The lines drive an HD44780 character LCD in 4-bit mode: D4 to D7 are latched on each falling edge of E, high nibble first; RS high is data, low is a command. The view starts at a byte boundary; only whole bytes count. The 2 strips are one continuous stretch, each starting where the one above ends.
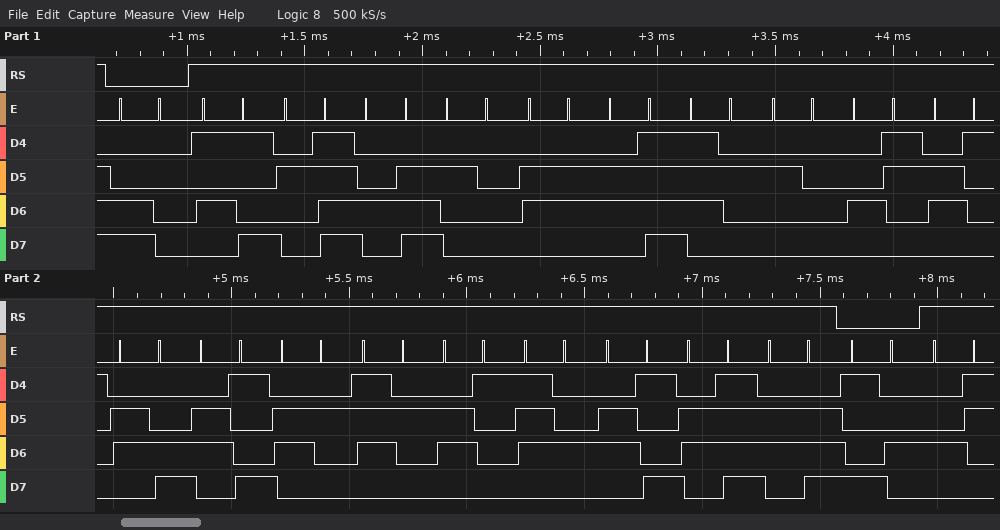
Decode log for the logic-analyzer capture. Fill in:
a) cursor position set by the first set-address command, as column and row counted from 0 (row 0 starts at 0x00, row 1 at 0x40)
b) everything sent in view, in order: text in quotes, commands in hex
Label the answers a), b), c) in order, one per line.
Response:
a) column 0, row 1
b) 0xC0 "Y/N for Calibration" 0x94 "C"
